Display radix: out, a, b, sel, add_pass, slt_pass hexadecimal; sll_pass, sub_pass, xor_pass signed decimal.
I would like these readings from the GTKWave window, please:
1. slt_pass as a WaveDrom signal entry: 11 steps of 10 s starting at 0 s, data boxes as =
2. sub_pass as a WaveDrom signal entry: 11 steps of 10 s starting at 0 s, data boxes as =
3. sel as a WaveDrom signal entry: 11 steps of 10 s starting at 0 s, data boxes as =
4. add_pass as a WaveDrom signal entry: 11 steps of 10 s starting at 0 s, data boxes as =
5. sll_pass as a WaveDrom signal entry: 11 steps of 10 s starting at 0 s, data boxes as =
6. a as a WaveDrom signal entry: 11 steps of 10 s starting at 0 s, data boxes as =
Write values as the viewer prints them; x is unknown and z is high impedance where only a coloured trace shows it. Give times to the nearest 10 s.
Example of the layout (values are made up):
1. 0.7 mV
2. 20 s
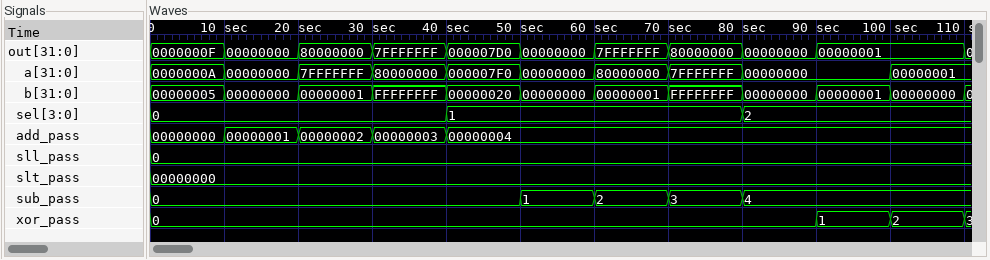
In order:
1. {name: 'slt_pass', wave: '=..........', data: '00000000'}
2. {name: 'sub_pass', wave: '=....====..', data: '0 1 2 3 4'}
3. {name: 'sel', wave: '=...=...=..', data: '0 1 2'}
4. {name: 'add_pass', wave: '=====......', data: '00000000 00000001 00000002 00000003 00000004'}
5. {name: 'sll_pass', wave: '=..........', data: '0'}
6. {name: 'a', wave: '=========.=', data: '0000000A 00000000 7FFFFFFF 80000000 000007F0 00000000 80000000 7FFFFFFF 00000000 00000001'}
